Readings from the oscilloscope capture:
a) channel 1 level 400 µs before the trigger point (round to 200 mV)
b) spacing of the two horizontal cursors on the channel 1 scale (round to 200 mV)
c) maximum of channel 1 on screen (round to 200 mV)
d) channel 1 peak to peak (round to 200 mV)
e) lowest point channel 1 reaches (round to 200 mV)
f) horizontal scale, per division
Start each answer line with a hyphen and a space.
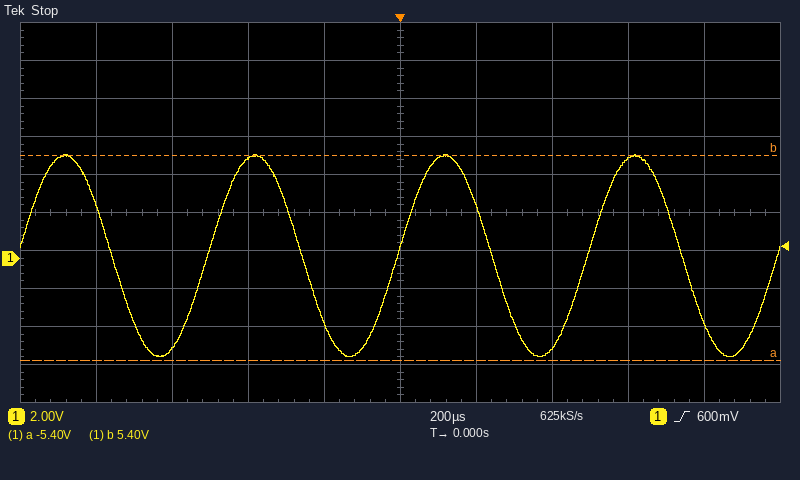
- 5.2 V
- 10.8 V
- 5.4 V
- 10.6 V
- -5.2 V
- 200 µs
